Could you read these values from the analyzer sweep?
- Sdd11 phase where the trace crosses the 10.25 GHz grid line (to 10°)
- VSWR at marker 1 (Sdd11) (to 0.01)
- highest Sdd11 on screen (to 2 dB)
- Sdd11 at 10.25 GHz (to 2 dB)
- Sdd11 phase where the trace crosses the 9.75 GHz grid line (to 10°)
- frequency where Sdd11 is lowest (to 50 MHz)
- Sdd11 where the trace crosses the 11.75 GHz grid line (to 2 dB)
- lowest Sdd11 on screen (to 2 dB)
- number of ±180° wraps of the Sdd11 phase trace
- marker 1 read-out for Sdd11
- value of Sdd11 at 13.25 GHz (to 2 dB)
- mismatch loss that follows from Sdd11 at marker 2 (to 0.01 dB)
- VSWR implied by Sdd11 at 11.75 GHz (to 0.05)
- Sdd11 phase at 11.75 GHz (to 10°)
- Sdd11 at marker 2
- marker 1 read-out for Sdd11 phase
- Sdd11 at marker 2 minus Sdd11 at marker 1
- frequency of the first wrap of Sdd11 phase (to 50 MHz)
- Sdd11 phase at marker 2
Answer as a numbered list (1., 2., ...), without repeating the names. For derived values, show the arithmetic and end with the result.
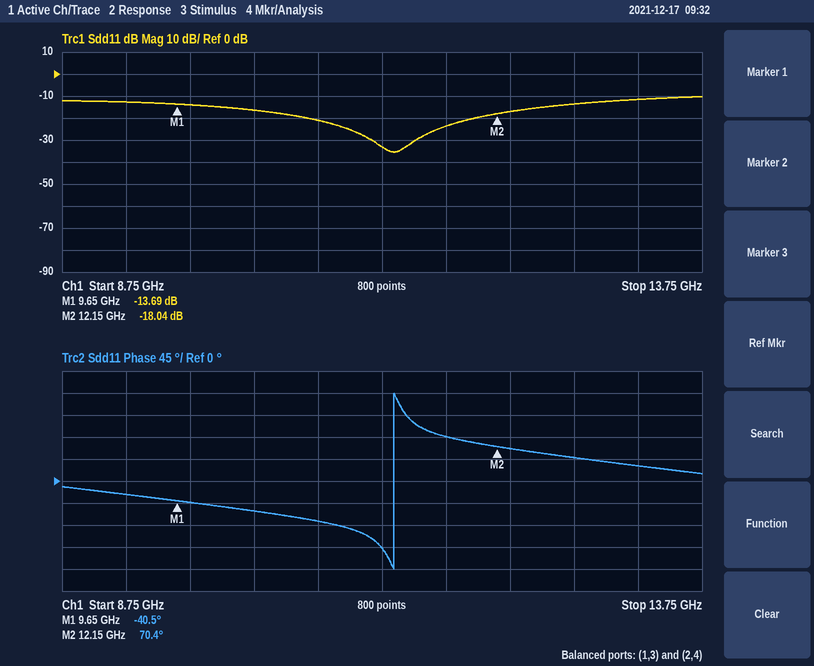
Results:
1. -60°
2. (1 + 0.2068)/(1 − 0.2068) ≈ 1.52
3. -10 dB
4. -16 dB
5. -40°
6. 11.35 GHz
7. -24 dB
8. -36 dB
9. 1
10. -13.69 dB
11. -12 dB
12. −10 log10(1 − 10^(-18.04/10)) ≈ 0.07 dB
13. |Γ| = 10^(-24/20) = 0.0631; VSWR = (1 + 0.0631)/(1 − 0.0631) ≈ 1.13, so 1.15 to the nearest 0.05
14. 90°
15. -18.04 dB
16. -40.5°
17. -18.04 − (-13.69) = -4.35 dB
18. 11.35 GHz
19. 70.4°
